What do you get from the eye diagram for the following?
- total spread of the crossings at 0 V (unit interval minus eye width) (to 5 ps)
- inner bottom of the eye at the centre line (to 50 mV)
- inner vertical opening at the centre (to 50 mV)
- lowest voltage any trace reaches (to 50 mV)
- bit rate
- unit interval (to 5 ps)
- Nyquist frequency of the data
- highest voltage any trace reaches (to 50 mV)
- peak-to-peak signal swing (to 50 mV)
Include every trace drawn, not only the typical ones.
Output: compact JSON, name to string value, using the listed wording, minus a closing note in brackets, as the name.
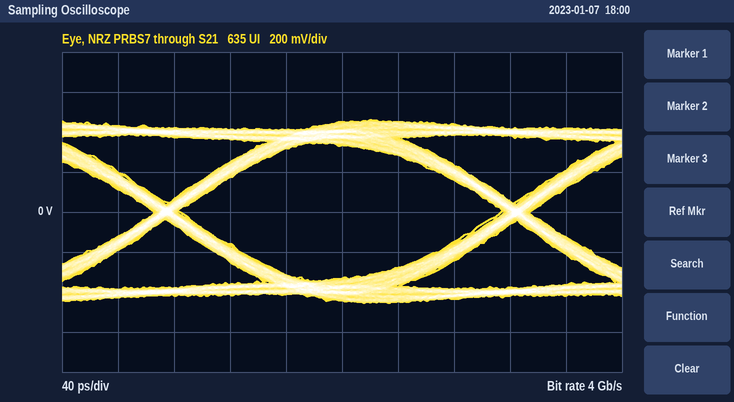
{"total spread of the crossings at 0 V (unit interval minus eye width)": "20 ps", "inner bottom of the eye at the centre line": "-350 mV", "inner vertical opening at the centre": "650 mV", "lowest voltage any trace reaches": "-450 mV", "bit rate": "4 Gb/s", "unit interval": "250 ps", "Nyquist frequency of the data": "2 GHz", "highest voltage any trace reaches": "450 mV", "peak-to-peak signal swing": "900 mV"}
